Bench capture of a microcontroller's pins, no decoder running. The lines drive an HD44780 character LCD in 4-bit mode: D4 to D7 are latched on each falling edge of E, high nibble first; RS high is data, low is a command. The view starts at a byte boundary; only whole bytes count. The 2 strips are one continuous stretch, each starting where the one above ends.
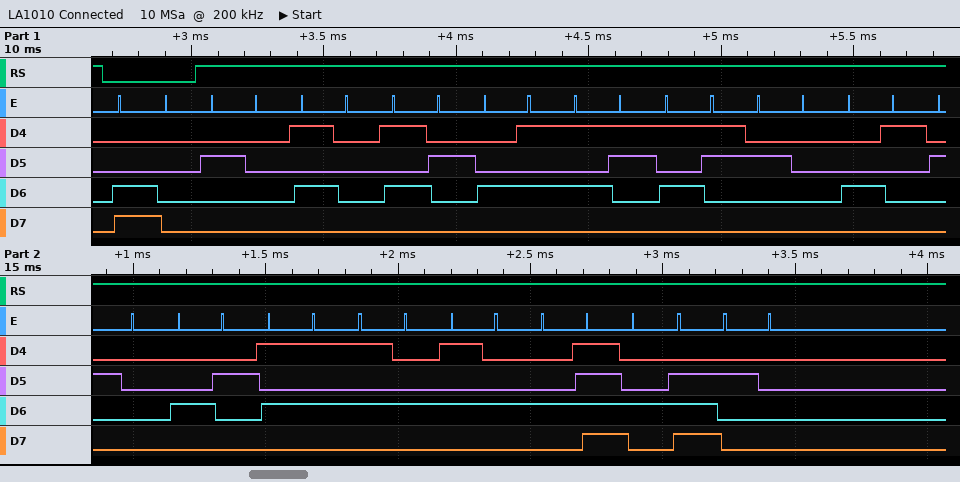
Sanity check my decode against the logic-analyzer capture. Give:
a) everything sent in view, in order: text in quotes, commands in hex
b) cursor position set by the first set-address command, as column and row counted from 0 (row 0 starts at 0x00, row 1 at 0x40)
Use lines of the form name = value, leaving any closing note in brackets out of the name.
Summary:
everything sent in view, in order: text in quotes, commands in hex = 0xC0 " PRESS A BUTTON "
cursor position set by the first set-address command, as column and row counted from 0 = column 0, row 1
